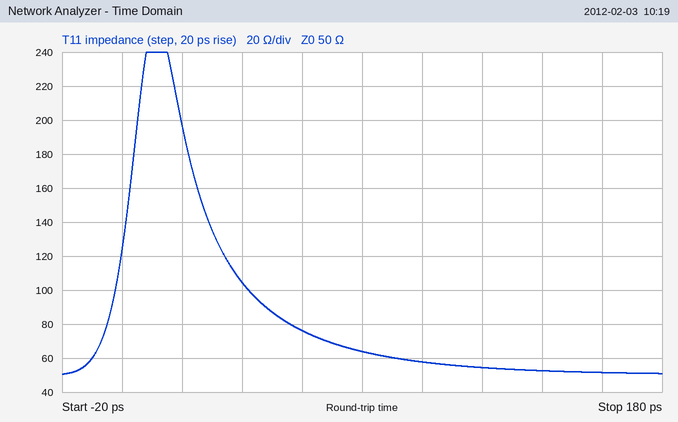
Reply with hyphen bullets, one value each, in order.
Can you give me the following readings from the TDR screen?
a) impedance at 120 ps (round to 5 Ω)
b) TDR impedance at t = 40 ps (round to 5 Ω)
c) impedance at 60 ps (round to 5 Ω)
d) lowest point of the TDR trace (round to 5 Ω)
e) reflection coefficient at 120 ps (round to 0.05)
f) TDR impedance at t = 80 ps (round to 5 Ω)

- 55 Ω
- 105 Ω
- 75 Ω
- 50 Ω
- +0.05
- 65 Ω
